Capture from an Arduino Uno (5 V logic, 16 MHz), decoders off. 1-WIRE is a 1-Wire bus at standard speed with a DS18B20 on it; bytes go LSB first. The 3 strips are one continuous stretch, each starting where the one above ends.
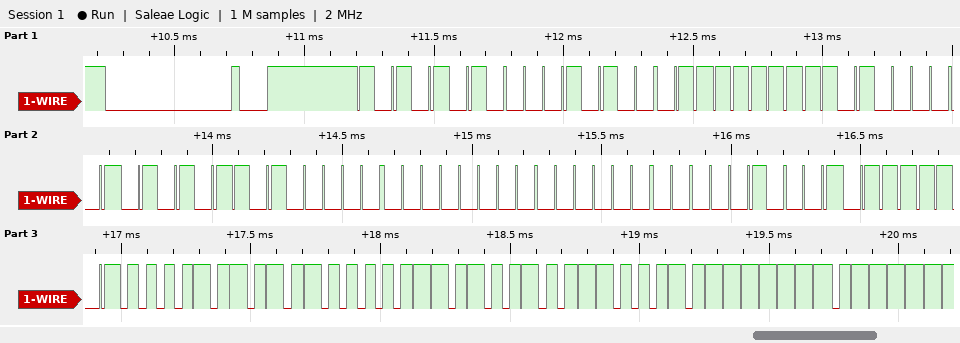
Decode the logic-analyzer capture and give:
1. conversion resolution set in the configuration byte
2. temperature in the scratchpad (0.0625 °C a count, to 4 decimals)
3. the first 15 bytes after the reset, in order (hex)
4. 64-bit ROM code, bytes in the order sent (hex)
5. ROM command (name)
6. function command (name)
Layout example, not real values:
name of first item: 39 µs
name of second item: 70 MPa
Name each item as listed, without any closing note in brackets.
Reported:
conversion resolution set in the configuration byte: 12 bits
temperature in the scratchpad: 85.0000 °C
the first 15 bytes after the reset, in order: 55 28 FE 0B AA 05 00 00 88 BE 50 05 4B 46 7F
64-bit ROM code, bytes in the order sent: 28 FE 0B AA 05 00 00 88
ROM command: Match ROM
function command: Read Scratchpad
